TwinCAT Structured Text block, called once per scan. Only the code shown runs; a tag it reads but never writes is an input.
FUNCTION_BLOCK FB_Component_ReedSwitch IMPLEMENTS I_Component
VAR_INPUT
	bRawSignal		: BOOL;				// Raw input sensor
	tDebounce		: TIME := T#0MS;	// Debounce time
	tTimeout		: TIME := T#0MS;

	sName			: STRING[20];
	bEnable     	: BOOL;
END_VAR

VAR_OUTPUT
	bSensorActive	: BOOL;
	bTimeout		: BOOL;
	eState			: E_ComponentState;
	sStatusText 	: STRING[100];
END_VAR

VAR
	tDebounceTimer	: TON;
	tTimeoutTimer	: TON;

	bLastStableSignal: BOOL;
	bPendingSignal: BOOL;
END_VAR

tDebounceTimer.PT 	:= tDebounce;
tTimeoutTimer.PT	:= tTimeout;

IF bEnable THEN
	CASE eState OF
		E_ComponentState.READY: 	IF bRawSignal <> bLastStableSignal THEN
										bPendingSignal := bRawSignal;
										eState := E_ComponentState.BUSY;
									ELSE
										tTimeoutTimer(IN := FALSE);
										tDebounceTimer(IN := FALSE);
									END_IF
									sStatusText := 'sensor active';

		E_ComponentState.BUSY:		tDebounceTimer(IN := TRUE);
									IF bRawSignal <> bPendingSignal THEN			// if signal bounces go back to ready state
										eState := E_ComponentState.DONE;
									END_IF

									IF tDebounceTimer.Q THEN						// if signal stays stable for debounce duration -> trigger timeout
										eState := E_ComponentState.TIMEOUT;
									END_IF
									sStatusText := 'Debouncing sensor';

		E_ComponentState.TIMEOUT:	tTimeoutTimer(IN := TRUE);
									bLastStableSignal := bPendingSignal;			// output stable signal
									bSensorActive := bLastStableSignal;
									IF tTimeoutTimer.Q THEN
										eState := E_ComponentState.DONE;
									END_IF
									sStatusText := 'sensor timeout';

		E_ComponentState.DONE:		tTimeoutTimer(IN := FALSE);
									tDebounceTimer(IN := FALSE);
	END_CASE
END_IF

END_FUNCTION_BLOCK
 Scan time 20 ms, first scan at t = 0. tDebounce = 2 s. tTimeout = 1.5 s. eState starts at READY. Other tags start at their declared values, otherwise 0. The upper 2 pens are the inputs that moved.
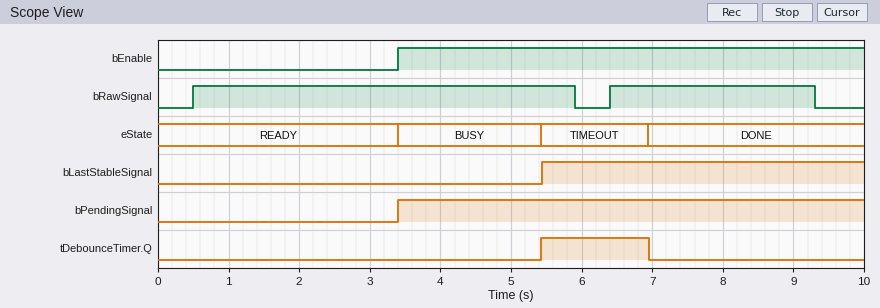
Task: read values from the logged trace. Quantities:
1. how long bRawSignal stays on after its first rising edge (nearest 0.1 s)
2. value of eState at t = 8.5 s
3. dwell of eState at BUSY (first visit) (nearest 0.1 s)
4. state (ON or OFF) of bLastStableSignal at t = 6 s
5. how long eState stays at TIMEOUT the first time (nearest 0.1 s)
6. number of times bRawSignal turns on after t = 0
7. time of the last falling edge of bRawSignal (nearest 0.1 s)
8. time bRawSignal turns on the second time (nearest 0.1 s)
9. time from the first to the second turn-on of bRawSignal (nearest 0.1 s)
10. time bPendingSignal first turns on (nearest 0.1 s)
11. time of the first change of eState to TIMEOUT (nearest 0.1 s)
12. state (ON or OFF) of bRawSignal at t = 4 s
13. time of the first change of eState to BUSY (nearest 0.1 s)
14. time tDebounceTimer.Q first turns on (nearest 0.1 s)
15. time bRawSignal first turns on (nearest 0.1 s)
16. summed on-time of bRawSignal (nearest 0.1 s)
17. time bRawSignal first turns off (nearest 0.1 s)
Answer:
5.4 s
DONE
2.0 s
ON
1.5 s
2
9.3 s
6.4 s
5.9 s
3.4 s
5.4 s
ON
3.4 s
5.4 s
0.5 s
8.3 s
5.9 s
